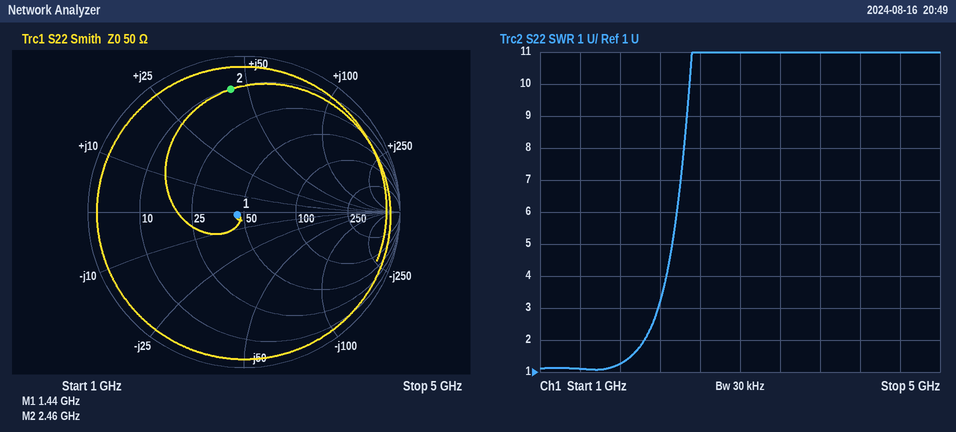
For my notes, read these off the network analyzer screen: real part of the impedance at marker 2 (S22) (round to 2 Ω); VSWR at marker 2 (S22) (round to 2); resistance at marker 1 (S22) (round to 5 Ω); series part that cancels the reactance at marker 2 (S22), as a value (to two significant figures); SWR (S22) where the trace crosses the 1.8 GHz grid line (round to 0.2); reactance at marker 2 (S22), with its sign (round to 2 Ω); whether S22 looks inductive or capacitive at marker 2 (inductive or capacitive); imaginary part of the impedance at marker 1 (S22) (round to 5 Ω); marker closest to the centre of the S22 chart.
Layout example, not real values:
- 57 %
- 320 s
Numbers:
- 10 Ω
- 8
- 45 Ω
- 1.5 pF
- 1.2
- +44 Ω
- inductive
- 0 Ω
- marker 1
